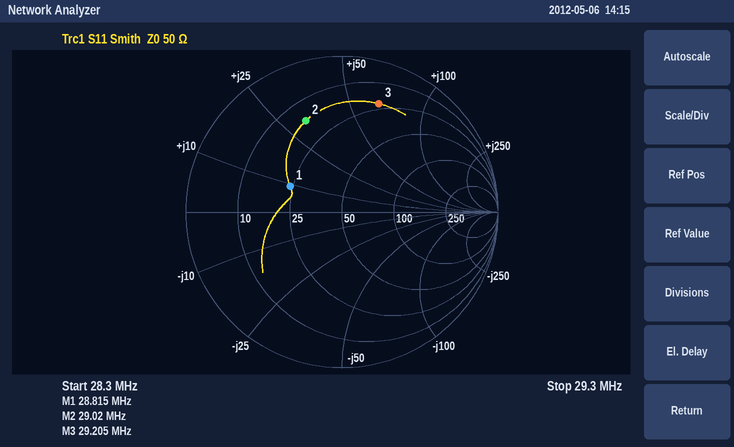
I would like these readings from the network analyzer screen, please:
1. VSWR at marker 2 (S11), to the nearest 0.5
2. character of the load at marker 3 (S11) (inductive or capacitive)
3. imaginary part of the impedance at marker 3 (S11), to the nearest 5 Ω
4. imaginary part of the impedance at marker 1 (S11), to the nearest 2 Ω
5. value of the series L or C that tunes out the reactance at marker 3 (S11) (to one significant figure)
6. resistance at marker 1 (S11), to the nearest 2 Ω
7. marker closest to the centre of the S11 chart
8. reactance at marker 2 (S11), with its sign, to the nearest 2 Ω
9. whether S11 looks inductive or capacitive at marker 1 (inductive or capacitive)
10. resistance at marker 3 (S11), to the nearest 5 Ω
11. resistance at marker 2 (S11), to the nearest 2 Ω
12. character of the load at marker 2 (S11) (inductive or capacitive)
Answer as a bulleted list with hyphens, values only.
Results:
- 4.5
- inductive
- +65 Ω
- +10 Ω
- 80 pF
- 24 Ω
- marker 1
- +32 Ω
- inductive
- 20 Ω
- 16 Ω
- inductive
